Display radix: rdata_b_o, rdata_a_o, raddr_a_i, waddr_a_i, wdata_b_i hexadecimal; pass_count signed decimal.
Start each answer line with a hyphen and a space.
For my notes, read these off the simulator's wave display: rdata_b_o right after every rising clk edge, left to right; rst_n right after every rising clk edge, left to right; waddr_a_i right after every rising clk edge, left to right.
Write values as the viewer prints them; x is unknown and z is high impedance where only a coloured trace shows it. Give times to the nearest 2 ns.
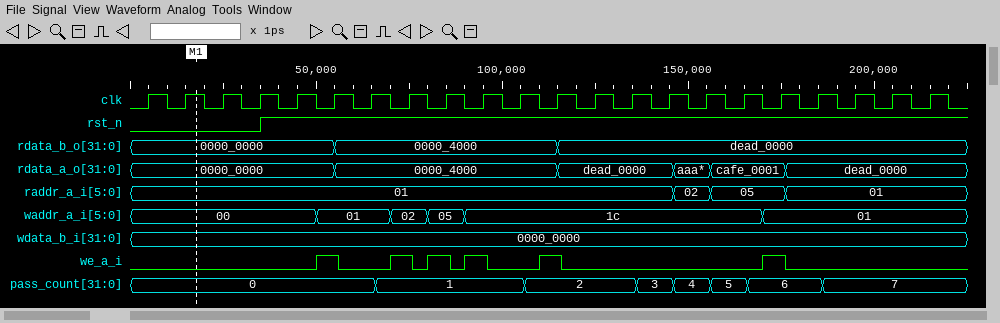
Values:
- 0000_0000, 0000_0000, 0000_0000, 0000_0000, 0000_0000, 0000_4000, 0000_4000, 0000_4000, 0000_4000, 0000_4000, 0000_4000, dead_0000, dead_0000, dead_0000, dead_0000, dead_0000, dead_0000, dead_0000, dead_0000, dead_0000, dead_0000, dead_0000
- 0 0 0 1 1 1 1 1 1 1 1 1 1 1 1 1 1 1 1 1 1 1
- 00, 00, 00, 00, 00, 01, 01, 02, 05, 1c, 1c, 1c, 1c, 1c, 1c, 1c, 1c, 01, 01, 01, 01, 01
